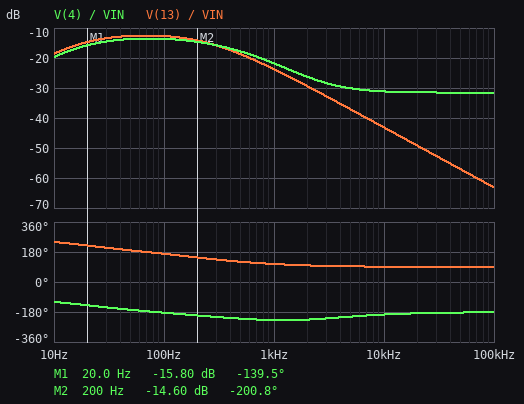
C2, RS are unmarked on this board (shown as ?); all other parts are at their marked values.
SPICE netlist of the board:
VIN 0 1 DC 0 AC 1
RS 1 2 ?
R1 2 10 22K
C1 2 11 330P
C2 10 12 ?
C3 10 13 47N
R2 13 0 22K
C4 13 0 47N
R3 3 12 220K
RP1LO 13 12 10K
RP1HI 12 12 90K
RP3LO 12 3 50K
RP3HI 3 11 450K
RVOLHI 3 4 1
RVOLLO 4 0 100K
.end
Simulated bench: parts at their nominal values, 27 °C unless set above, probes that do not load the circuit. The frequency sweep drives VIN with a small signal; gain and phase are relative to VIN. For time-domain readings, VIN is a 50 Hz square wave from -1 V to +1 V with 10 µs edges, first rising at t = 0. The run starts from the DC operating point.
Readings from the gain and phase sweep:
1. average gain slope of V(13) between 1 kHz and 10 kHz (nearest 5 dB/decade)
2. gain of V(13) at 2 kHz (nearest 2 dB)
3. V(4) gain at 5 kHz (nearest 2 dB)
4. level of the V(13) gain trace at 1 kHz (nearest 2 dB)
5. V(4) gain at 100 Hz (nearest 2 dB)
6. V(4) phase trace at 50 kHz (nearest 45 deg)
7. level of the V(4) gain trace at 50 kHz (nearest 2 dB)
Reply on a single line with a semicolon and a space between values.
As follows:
-20 dB/decade; -30 dB; -30 dB; -24 dB; -14 dB; -180 deg; -32 dB
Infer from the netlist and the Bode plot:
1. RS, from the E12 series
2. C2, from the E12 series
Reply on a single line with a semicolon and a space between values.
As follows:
27 kΩ; 68 nF
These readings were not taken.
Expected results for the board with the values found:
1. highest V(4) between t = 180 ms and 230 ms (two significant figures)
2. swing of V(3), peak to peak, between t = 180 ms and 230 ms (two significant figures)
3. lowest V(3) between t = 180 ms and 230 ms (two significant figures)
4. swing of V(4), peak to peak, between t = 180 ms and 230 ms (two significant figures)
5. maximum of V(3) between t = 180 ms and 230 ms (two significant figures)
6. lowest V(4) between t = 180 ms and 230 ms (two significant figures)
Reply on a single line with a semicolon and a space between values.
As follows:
280 mV; 560 mV; -280 mV; 560 mV; 280 mV; -280 mV
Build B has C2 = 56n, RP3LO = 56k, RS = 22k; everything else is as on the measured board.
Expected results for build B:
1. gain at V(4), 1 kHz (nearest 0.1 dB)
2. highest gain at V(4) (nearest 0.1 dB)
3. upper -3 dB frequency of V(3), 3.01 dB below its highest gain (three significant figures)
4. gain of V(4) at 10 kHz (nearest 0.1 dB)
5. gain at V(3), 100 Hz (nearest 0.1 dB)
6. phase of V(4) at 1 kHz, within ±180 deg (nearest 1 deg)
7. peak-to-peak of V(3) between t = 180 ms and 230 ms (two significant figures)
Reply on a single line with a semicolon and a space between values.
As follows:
-21.2 dB; -13.3 dB; 387 Hz; -29.7 dB; -13.4 dB; 134 deg; 590 mV
